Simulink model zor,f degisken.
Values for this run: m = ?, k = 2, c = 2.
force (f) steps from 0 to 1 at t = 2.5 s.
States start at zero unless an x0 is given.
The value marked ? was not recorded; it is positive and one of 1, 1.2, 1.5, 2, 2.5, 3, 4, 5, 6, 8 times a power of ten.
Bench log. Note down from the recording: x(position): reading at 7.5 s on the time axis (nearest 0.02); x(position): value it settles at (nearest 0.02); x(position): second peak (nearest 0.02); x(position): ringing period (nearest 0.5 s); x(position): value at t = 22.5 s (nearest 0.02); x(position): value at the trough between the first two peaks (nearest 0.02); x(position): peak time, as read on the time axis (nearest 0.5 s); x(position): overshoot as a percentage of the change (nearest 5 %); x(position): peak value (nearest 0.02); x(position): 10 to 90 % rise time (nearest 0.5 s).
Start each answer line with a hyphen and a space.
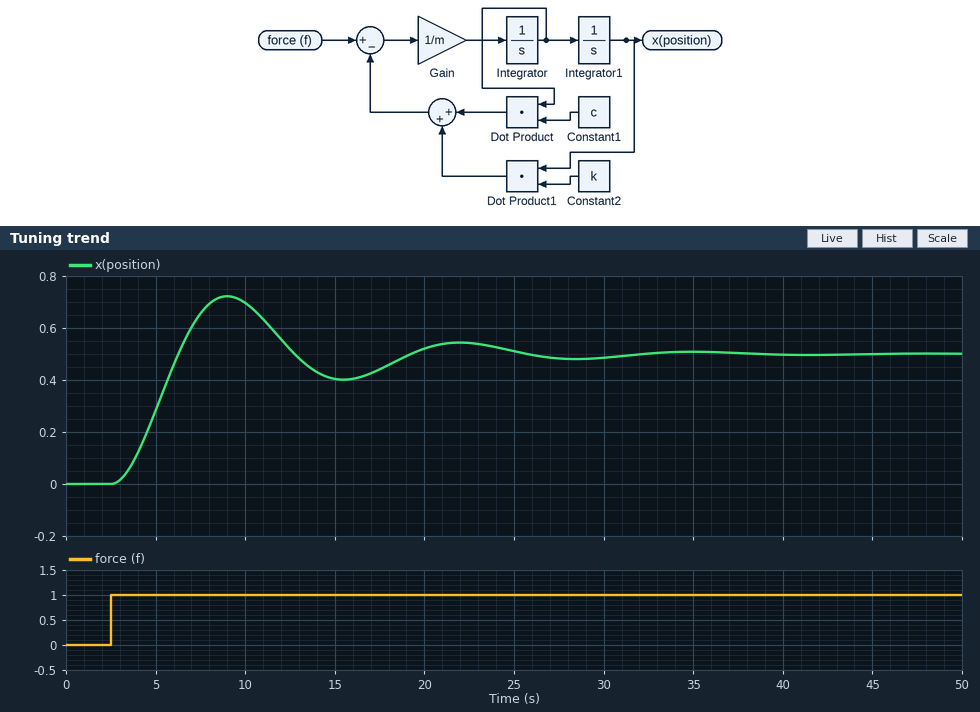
- 0.66
- 0.50
- 0.54
- 13.0 s
- 0.54
- 0.40
- 9.0 s
- 45 %
- 0.72
- 2.5 s
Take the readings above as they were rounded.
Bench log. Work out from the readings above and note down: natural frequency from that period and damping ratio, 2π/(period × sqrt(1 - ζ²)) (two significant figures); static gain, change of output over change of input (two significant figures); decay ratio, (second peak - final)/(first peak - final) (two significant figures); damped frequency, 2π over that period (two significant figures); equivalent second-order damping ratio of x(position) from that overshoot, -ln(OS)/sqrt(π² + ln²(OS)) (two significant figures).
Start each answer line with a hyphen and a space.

- 0.50 rad/s
- 0.50
- 0.18
- 0.48 rad/s
- 0.25
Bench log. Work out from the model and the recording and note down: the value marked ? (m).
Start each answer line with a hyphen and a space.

- 8
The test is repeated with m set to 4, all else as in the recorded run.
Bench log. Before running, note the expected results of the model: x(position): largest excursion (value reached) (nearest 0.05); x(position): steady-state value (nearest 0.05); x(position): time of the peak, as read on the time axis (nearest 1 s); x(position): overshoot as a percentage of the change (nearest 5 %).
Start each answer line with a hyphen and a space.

- 0.65
- 0.50
- 7 s
- 30 %
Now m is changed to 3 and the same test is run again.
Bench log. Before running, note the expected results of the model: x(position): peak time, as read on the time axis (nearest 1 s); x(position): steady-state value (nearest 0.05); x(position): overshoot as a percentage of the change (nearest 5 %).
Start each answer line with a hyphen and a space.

- 7 s
- 0.50
- 25 %
